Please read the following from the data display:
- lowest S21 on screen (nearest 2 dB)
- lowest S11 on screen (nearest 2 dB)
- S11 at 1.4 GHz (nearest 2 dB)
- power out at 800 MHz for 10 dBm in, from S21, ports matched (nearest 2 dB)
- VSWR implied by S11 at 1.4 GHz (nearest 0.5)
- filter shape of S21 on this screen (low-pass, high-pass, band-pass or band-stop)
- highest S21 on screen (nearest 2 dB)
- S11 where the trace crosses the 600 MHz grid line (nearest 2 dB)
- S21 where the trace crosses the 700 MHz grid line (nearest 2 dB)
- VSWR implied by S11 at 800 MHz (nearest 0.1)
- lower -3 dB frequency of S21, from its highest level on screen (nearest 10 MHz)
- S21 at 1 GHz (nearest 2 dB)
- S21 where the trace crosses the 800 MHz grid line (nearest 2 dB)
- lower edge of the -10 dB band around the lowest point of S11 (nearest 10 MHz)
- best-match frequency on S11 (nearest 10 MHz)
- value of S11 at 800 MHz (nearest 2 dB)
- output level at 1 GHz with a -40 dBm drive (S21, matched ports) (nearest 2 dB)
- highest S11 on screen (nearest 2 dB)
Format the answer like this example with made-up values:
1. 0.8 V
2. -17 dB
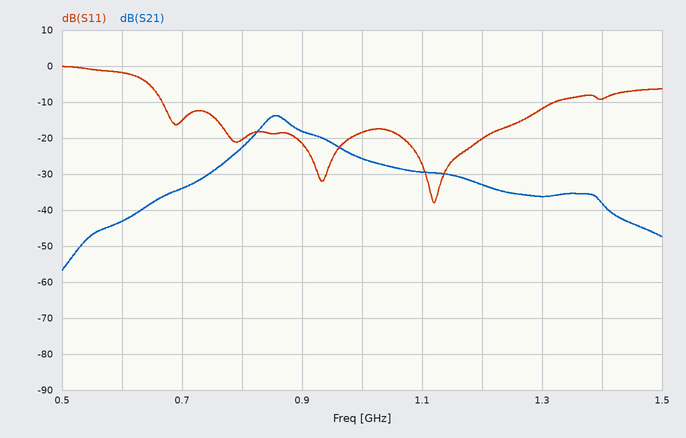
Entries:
1. -56 dB
2. -38 dB
3. -10 dB
4. -12 dBm
5. 2.0
6. band-pass
7. -14 dB
8. -2 dB
9. -34 dB
10. 1.2
11. 830 MHz
12. -26 dB
13. -22 dB
14. 670 MHz
15. 1.12 GHz
16. -20 dB
17. -66 dBm
18. 0 dB
